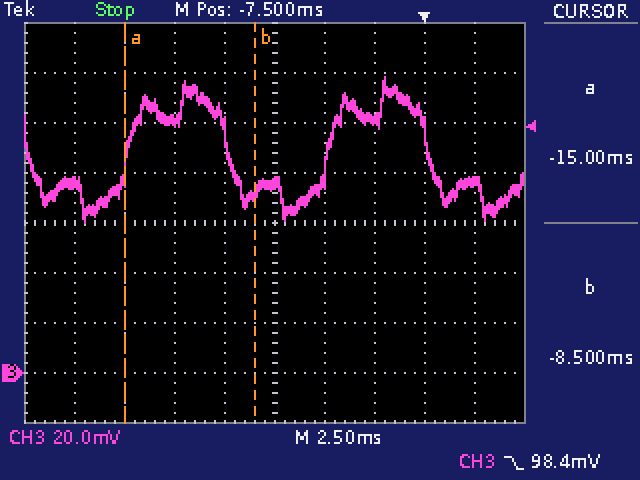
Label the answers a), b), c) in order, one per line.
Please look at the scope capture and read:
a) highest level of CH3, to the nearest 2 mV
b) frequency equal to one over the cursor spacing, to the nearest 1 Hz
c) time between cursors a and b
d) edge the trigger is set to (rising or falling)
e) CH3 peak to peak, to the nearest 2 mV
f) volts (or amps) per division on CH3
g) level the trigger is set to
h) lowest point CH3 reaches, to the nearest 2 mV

a) 118 mV
b) 154 Hz
c) 6.50 ms
d) falling
e) 58 mV
f) 20 mV
g) 98.4 mV
h) 60 mV
